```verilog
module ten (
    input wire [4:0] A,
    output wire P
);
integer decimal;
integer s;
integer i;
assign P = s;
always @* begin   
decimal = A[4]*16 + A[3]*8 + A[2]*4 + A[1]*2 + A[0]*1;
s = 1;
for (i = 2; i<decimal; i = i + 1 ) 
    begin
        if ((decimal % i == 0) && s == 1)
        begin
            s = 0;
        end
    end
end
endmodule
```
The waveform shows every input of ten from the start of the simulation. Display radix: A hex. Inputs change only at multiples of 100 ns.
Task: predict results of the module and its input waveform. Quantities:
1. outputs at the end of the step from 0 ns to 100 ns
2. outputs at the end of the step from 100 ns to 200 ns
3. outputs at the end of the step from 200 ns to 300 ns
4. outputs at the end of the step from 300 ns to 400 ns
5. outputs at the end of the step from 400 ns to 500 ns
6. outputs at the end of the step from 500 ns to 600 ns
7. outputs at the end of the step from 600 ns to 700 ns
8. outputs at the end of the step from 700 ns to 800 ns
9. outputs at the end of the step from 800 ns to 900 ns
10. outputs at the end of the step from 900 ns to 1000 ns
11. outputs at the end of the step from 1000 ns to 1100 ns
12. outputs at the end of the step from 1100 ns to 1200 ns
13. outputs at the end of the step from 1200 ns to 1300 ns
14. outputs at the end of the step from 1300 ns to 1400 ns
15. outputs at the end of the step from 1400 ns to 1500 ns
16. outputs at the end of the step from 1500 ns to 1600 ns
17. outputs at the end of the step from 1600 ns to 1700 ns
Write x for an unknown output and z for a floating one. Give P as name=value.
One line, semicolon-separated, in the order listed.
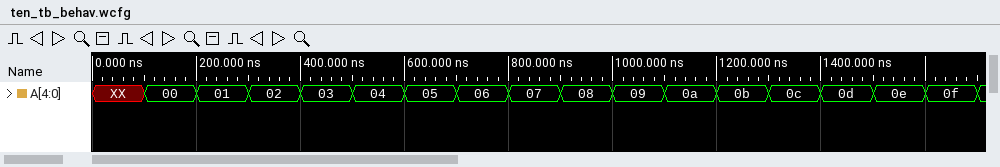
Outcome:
P=x; P=1; P=1; P=1; P=1; P=0; P=1; P=0; P=1; P=0; P=0; P=0; P=1; P=0; P=1; P=0; P=0
